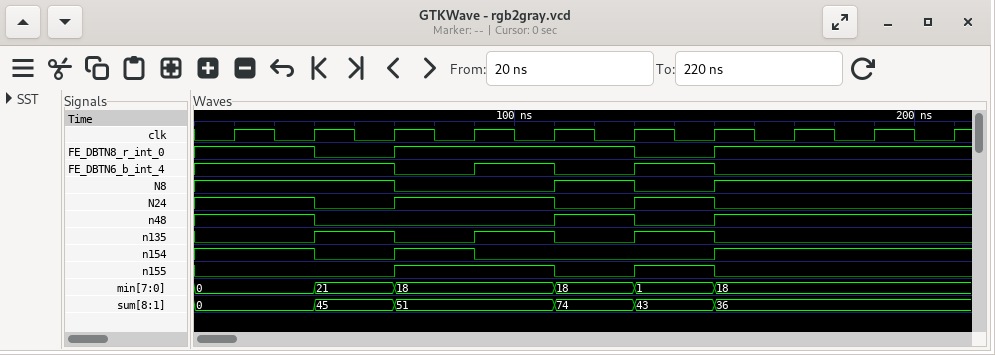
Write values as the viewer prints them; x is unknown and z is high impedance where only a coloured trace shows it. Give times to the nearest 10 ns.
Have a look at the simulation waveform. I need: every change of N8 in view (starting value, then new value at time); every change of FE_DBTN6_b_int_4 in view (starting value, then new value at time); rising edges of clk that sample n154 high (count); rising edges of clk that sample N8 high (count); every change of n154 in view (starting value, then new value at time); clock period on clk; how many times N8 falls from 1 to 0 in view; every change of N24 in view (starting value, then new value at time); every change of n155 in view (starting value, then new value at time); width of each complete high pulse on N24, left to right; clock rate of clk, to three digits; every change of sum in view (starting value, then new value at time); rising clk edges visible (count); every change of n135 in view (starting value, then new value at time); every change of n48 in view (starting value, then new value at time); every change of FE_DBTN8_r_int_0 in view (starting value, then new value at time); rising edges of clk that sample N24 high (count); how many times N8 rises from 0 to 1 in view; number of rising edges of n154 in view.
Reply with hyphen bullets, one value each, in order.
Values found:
- 1, 0 at 70 ns, 1 at 110 ns, 0 at 130 ns, 1 at 150 ns
- 1, 0 at 70 ns, 1 at 90 ns, 0 at 110 ns, 1 at 130 ns, 0 at 150 ns
- 6
- 7
- 1, 0 at 50 ns, 1 at 70 ns, 0 at 90 ns, 1 at 150 ns
- 20 ns
- 2
- 1, 0 at 50 ns, 1 at 70 ns, 0 at 110 ns, 1 at 130 ns, 0 at 150 ns
- 0, 1 at 70 ns, 0 at 110 ns, 1 at 130 ns, 0 at 150 ns
- 40 ns, 20 ns
- 50.0 MHz
- 0, 45 at 50 ns, 51 at 70 ns, 74 at 110 ns, 43 at 130 ns, 36 at 150 ns
- 10
- 0, 1 at 50 ns, 0 at 70 ns, 1 at 90 ns, 0 at 110 ns, 1 at 130 ns, 0 at 150 ns
- 1, 0 at 50 ns, 1 at 110 ns, 0 at 130 ns, 1 at 150 ns
- 1, 0 at 50 ns, 1 at 70 ns, 0 at 130 ns, 1 at 150 ns
- 5
- 2
- 2
